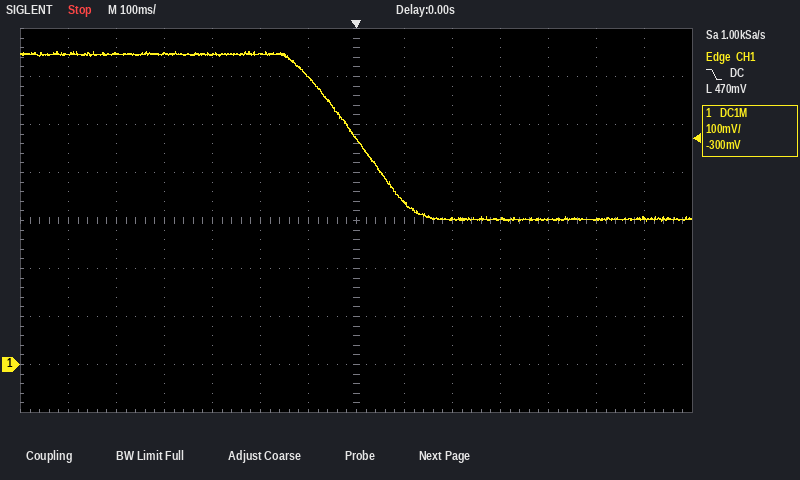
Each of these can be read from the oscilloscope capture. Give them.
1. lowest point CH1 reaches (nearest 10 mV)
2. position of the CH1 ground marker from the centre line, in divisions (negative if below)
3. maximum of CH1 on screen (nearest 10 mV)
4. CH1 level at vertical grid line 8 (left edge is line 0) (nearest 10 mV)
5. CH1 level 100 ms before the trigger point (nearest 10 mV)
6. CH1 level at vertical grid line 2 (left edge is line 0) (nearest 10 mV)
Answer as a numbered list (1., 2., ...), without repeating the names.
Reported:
1. 300 mV
2. -3.0 div
3. 650 mV
4. 340 mV
5. 600 mV
6. 650 mV
